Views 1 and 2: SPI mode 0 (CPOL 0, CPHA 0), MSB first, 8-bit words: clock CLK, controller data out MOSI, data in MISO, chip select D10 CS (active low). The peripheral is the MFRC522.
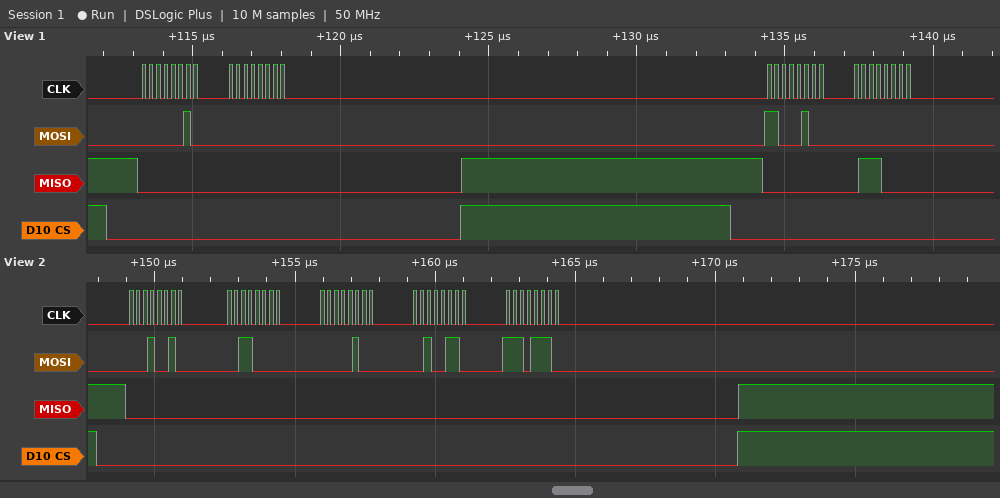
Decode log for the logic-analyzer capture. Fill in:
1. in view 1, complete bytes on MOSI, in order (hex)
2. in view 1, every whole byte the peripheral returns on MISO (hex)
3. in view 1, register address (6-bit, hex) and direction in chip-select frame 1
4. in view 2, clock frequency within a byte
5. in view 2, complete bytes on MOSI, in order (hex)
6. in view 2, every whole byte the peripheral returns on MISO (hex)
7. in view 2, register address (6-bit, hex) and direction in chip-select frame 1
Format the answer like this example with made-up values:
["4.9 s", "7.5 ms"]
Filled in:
["0x02 0x00 0xC4 0x00", "0x00 0x00 0x00 0x70", "0x01 write", "4 MHz", "12 30 04 26 EE", "00 00 00 00 00", "0x09 write"]
